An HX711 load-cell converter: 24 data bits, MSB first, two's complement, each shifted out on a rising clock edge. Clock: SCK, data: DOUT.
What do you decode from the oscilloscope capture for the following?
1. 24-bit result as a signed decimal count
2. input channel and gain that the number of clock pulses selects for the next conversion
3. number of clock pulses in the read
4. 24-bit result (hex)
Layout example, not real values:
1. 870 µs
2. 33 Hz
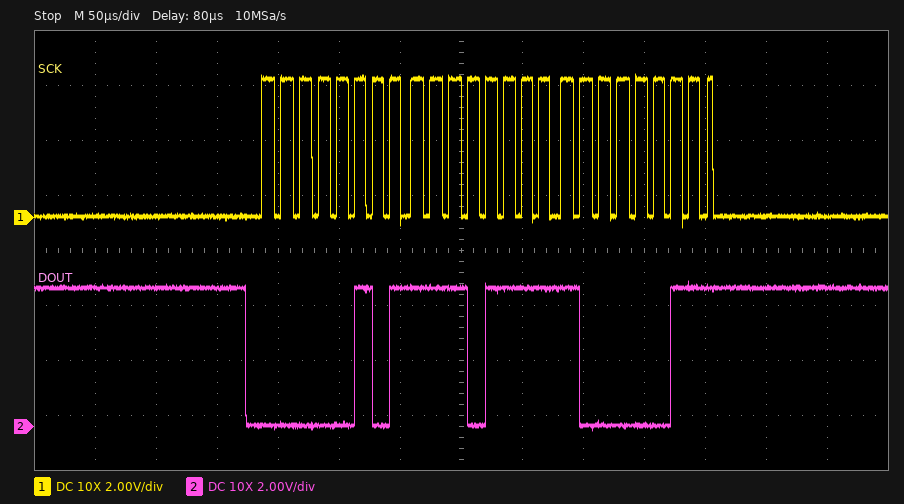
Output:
1. 388995
2. channel A, gain 128
3. 25
4. 0x05EF83
